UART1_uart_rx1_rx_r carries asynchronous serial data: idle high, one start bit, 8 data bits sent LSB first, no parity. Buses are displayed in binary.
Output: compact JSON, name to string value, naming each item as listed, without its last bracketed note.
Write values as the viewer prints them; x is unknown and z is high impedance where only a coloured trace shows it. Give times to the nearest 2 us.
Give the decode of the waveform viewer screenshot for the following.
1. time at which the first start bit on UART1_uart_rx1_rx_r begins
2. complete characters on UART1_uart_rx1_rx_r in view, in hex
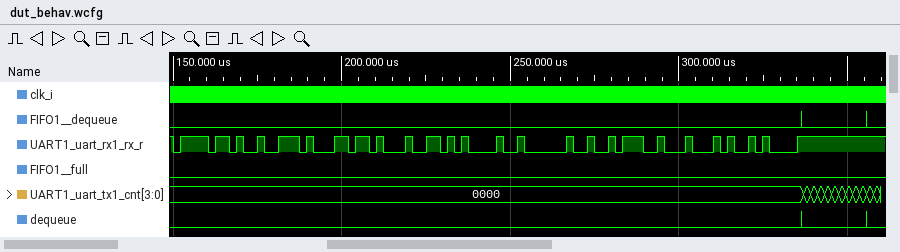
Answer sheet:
{"time at which the first start bit on UART1_uart_rx1_rx_r begins": "150 us", "complete characters on UART1_uart_rx1_rx_r in view, in hex": "6F, 72, 6C, 64, 21, 20, 3A, 44, 0A"}
